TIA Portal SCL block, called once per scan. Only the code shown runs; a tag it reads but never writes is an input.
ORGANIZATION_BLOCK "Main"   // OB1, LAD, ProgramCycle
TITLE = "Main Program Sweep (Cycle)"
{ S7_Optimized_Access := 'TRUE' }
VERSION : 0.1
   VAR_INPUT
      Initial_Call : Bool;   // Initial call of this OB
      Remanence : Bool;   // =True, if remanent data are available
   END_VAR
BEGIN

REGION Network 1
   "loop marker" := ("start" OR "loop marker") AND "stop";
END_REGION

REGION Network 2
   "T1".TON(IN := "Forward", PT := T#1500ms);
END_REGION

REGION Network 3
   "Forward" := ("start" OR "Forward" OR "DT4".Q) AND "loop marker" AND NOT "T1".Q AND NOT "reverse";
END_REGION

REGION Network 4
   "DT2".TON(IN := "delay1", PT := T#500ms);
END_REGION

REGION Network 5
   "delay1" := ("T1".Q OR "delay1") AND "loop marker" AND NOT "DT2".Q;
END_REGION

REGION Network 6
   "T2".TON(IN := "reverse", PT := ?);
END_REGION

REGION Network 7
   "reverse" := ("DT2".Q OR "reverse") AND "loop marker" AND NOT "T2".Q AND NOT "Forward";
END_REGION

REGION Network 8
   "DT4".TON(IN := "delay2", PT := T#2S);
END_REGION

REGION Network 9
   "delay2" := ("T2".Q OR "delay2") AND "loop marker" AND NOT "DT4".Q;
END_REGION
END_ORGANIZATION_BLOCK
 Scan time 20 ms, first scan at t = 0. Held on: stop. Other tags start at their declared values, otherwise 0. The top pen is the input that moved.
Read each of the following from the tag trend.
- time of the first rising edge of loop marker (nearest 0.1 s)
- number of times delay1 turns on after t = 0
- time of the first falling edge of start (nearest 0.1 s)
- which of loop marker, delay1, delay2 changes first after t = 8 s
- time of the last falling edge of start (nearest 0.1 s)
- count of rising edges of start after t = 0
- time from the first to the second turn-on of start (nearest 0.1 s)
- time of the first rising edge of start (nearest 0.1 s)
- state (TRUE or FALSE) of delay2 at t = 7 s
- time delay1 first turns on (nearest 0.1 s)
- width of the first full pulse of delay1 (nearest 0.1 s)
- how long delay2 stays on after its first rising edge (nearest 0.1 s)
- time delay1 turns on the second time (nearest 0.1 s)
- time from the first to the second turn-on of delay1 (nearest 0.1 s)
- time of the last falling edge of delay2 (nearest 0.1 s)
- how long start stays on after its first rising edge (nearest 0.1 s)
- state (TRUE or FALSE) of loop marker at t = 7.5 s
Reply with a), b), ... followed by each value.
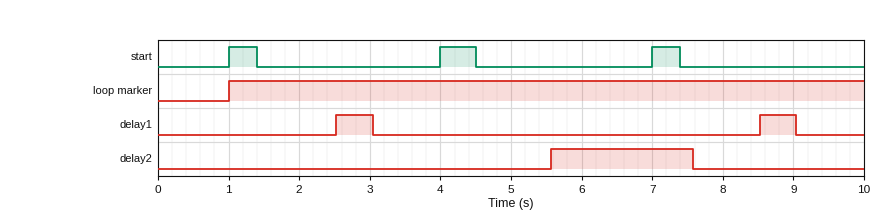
a) 1.0 s
b) 2
c) 1.4 s
d) delay1
e) 7.4 s
f) 3
g) 3.0 s
h) 1.0 s
i) TRUE
j) 2.5 s
k) 0.5 s
l) 2.0 s
m) 8.5 s
n) 6.0 s
o) 7.6 s
p) 0.4 s
q) TRUE
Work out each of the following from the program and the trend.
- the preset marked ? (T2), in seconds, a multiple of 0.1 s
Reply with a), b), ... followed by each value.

a) 2.5 s
